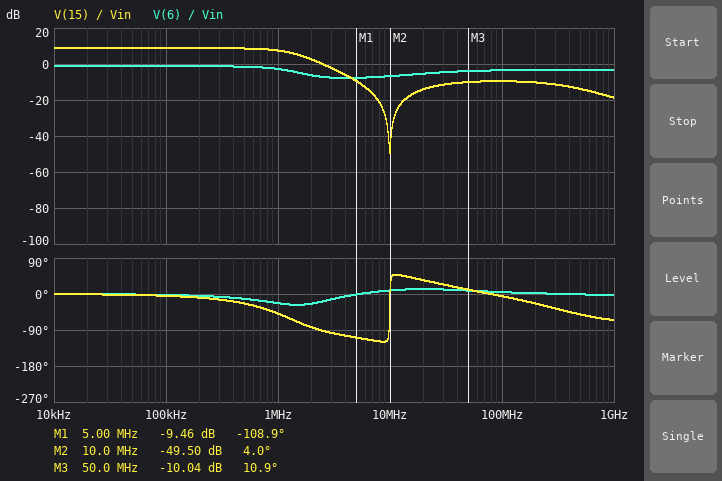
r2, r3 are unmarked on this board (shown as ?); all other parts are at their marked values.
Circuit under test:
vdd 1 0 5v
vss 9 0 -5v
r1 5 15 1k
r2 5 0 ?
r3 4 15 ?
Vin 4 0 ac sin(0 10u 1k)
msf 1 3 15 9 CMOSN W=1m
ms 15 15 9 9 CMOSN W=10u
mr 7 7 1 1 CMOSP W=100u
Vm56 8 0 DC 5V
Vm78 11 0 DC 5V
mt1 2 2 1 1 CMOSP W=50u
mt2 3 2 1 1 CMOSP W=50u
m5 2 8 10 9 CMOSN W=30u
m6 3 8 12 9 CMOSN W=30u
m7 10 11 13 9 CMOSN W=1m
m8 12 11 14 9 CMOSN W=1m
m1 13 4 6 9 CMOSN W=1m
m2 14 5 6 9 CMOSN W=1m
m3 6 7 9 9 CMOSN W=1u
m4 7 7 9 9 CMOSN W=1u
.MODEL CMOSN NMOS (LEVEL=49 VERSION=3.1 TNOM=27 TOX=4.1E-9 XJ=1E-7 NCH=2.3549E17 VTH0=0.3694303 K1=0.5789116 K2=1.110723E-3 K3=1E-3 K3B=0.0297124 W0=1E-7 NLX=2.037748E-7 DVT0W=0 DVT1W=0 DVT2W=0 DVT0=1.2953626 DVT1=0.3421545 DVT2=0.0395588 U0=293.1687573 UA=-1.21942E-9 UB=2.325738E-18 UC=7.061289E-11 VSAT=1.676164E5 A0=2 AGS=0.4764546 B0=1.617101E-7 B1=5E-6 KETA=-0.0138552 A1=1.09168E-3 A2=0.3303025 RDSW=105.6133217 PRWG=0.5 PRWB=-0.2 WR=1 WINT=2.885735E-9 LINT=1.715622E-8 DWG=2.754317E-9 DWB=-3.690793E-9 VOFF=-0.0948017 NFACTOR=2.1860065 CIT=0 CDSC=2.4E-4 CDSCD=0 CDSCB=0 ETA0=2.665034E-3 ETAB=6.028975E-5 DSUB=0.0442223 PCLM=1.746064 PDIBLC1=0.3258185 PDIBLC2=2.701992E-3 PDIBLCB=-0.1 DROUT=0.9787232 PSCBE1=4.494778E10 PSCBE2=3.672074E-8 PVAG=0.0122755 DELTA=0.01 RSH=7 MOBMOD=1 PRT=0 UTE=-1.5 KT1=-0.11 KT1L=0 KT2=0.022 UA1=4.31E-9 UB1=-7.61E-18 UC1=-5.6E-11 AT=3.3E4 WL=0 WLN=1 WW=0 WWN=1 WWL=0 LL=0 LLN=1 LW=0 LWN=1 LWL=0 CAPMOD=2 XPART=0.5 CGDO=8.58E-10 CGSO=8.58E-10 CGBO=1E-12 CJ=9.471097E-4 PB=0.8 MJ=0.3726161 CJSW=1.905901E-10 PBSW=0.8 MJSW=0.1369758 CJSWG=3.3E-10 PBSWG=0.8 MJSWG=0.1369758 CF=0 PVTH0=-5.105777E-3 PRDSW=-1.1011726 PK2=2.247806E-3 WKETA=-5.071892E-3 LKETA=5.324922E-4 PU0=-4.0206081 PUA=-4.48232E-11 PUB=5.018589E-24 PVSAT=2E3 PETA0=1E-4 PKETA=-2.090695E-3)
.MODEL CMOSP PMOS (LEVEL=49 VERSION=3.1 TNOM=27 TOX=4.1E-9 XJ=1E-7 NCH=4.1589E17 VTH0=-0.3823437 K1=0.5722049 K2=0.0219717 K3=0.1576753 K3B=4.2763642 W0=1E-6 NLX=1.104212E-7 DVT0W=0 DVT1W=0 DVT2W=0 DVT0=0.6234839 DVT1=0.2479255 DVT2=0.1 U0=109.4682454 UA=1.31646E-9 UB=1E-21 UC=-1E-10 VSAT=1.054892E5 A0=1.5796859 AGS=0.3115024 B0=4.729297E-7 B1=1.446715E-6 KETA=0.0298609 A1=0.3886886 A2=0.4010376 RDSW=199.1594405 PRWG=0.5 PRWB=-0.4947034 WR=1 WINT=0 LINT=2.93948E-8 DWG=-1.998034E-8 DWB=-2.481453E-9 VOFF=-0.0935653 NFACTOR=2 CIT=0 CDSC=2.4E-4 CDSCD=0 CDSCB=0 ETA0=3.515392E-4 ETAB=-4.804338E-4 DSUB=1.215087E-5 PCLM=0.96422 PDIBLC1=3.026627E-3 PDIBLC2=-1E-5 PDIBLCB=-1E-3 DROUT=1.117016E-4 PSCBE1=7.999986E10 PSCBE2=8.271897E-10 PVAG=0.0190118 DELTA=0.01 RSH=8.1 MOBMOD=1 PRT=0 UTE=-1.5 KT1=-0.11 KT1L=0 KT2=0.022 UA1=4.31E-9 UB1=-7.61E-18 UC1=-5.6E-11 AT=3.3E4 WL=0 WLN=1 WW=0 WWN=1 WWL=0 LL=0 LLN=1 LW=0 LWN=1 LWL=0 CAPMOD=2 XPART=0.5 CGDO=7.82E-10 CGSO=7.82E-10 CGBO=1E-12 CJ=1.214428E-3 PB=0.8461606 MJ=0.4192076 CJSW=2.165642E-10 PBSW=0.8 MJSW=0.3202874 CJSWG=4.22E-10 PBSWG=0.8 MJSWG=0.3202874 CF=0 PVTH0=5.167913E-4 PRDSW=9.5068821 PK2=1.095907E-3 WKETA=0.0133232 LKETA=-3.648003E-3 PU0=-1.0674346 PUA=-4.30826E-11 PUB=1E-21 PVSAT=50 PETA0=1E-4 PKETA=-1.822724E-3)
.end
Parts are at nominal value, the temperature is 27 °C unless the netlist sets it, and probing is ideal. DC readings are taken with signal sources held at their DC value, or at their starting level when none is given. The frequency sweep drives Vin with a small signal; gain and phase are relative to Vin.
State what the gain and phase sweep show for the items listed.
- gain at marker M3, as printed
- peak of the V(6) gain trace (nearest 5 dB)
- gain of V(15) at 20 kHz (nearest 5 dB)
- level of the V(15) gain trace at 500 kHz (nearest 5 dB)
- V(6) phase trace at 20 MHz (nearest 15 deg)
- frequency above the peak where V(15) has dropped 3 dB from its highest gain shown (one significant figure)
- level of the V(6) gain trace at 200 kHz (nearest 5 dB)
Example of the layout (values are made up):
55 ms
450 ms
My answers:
-10.04 dB
0 dB
10 dB
10 dB
15 deg
1 MHz
0 dB
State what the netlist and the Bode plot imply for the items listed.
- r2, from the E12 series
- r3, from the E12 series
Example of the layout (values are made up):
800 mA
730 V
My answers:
560 Ω
560 Ω
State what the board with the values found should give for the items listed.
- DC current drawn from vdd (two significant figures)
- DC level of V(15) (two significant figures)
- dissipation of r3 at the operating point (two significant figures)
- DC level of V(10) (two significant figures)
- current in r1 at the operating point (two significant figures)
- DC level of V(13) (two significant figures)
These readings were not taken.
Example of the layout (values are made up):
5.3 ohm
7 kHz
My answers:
3.1 mA
13 mV
310 nW
3.1 V
8.4 µA
3.1 V
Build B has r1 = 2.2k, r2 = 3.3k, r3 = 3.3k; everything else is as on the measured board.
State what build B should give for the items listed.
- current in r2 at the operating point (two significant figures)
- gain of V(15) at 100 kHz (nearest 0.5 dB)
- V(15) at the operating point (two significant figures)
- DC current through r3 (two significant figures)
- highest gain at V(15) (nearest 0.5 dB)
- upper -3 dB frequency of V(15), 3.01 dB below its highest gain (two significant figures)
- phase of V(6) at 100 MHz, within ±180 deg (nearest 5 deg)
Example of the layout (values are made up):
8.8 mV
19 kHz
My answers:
1.4 µA
4.5 dB
7.9 mV
2.4 µA
5.0 dB
2.7 MHz
0 deg
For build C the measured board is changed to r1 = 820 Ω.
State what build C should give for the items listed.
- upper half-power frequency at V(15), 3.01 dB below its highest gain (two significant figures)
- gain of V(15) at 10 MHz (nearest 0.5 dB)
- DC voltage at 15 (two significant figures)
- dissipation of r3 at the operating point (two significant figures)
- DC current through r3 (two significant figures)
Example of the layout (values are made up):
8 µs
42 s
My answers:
1.5 MHz
-50.5 dB
12 mV
240 nW
21 µA
